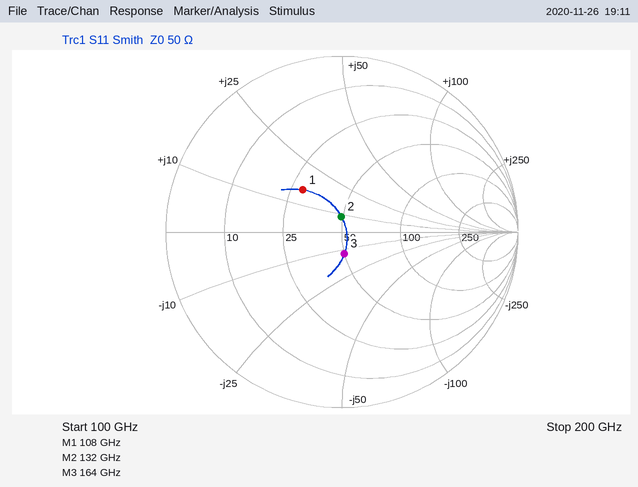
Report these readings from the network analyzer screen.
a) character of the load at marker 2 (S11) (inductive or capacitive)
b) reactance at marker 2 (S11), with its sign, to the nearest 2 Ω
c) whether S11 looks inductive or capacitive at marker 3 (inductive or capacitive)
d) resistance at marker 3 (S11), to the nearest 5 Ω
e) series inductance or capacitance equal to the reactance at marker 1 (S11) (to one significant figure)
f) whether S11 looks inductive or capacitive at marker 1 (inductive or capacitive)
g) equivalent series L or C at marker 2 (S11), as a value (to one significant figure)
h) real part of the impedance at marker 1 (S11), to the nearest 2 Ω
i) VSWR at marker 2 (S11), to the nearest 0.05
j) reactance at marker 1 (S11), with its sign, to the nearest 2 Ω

inductive
+8 Ω
capacitive
50 Ω
20 pH
inductive
10 pH
28 Ω
1.20
+16 Ω
